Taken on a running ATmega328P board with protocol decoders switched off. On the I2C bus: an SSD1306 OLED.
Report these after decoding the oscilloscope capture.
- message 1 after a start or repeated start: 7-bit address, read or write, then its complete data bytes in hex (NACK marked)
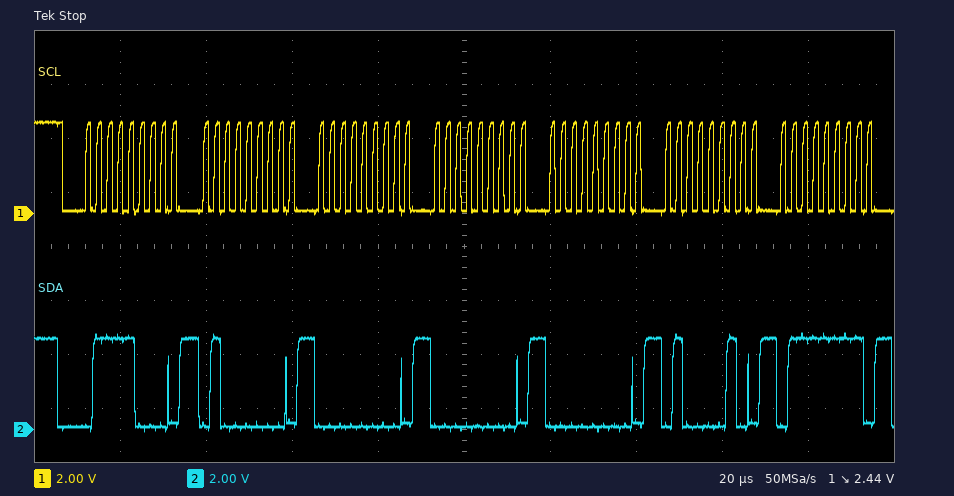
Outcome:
0x3C write: 40 00 00 00 42 7F
